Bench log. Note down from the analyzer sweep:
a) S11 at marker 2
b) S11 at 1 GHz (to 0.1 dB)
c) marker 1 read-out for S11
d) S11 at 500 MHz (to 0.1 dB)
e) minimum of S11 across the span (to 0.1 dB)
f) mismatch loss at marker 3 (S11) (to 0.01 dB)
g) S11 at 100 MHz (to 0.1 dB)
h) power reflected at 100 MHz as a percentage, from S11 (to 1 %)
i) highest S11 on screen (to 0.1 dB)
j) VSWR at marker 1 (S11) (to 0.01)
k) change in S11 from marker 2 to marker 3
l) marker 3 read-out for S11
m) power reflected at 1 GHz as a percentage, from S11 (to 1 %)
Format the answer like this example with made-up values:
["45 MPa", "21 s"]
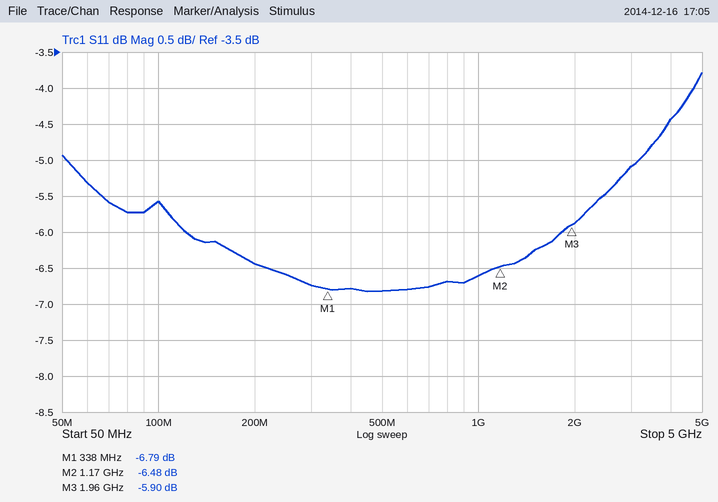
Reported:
["-6.48 dB", "-6.6 dB", "-6.79 dB", "-6.8 dB", "-6.8 dB", "1.29 dB", "-5.6 dB", "28 %", "-3.8 dB", "2.69", "0.58 dB", "-5.90 dB", "22 %"]
